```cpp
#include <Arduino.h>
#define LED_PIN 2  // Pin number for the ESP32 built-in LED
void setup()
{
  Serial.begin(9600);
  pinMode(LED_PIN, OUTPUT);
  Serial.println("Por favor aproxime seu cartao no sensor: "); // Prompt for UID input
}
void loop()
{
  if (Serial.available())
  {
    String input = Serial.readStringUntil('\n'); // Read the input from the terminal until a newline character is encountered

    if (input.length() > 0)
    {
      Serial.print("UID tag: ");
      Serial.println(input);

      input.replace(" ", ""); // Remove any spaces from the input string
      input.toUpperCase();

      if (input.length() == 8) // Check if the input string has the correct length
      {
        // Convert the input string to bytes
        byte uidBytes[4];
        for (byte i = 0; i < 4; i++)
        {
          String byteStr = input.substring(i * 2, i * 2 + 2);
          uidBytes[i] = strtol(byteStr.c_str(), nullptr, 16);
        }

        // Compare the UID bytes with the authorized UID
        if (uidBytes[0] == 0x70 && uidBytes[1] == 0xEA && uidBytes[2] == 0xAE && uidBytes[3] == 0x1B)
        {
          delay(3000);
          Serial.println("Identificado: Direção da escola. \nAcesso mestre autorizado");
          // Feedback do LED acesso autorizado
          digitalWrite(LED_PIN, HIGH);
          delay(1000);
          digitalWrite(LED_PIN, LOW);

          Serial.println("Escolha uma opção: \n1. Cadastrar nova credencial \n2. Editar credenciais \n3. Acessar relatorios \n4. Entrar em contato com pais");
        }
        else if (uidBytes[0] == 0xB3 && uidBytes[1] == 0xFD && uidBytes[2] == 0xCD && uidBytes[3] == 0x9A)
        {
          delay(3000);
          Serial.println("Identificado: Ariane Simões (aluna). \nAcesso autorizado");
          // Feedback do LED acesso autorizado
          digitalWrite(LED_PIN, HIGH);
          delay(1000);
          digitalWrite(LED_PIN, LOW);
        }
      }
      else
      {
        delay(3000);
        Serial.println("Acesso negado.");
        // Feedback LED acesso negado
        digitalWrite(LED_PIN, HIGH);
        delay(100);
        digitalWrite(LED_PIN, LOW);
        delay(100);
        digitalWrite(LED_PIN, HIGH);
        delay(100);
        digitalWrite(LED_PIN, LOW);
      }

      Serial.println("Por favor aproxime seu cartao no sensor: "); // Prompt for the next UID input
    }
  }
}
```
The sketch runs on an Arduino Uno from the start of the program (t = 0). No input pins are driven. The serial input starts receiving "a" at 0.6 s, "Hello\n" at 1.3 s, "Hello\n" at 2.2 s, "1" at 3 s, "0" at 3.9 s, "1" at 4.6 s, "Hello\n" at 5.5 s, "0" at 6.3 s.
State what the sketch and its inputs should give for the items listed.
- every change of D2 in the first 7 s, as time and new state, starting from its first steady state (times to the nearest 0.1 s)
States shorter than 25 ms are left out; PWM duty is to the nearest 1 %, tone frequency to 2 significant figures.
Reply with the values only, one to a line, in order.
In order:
0 s low; 4.3 s high; 4.4 s low; 4.5 s high; 4.6 s low
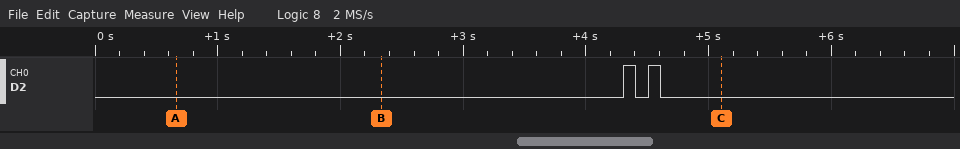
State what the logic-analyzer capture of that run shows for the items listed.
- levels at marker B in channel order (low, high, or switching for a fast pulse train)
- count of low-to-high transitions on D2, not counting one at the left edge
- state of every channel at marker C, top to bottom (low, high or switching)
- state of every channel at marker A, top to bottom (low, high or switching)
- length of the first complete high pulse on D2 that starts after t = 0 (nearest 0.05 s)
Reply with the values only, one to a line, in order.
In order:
D2 low
2
D2 low
D2 low
0.10 s
